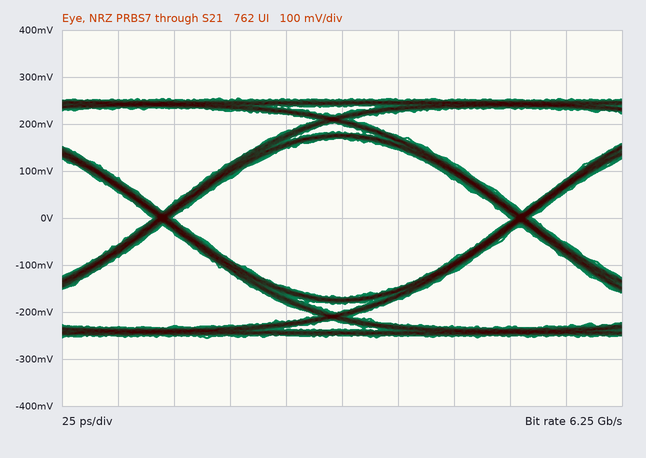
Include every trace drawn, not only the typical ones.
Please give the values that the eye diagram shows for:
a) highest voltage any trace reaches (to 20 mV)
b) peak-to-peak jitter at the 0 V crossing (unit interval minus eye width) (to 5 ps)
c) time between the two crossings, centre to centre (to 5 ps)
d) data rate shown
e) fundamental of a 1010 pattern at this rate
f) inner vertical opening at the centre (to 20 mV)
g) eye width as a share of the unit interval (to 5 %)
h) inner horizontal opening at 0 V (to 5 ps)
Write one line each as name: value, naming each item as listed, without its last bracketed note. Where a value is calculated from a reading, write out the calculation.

highest voltage any trace reaches: 260 mV
peak-to-peak jitter at the 0 V crossing (unit interval minus eye width): 10 ps
time between the two crossings, centre to centre: 160 ps
data rate shown: 6.25 Gb/s
fundamental of a 1010 pattern at this rate: 3.125 GHz
inner vertical opening at the centre: 340 mV
eye width as a share of the unit interval: 150 ps / 160 ps ≈ 93.8 %, so 95 % to the nearest 5 %
inner horizontal opening at 0 V: 150 ps
